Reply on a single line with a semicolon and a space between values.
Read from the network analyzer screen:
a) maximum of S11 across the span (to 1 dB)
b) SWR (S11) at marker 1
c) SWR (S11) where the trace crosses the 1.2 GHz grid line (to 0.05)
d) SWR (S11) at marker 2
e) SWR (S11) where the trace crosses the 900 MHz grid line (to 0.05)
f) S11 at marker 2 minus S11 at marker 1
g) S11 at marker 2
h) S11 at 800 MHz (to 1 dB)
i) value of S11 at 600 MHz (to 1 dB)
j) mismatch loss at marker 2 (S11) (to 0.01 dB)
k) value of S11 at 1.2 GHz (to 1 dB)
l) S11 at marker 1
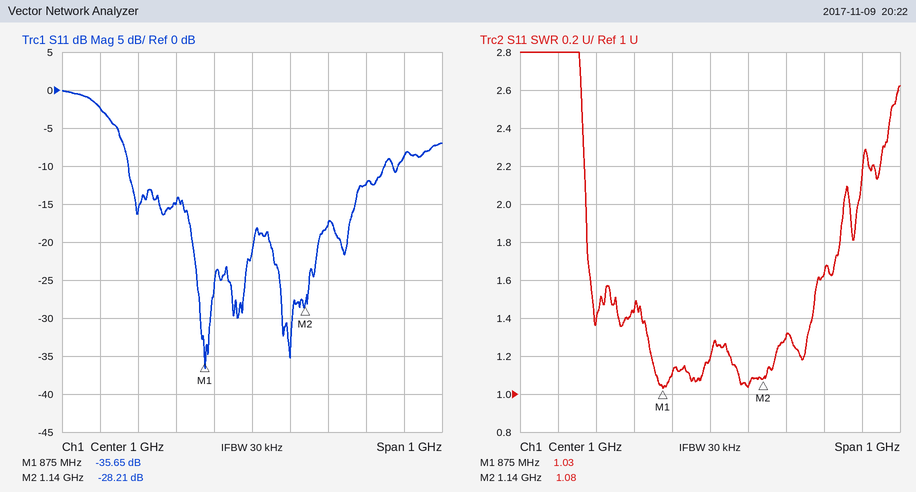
0 dB; 1.03; 1.30; 1.08; 1.10; 7.44 dB; -28.21 dB; -15 dB; -2 dB; 0.01 dB; -18 dB; -35.65 dB
